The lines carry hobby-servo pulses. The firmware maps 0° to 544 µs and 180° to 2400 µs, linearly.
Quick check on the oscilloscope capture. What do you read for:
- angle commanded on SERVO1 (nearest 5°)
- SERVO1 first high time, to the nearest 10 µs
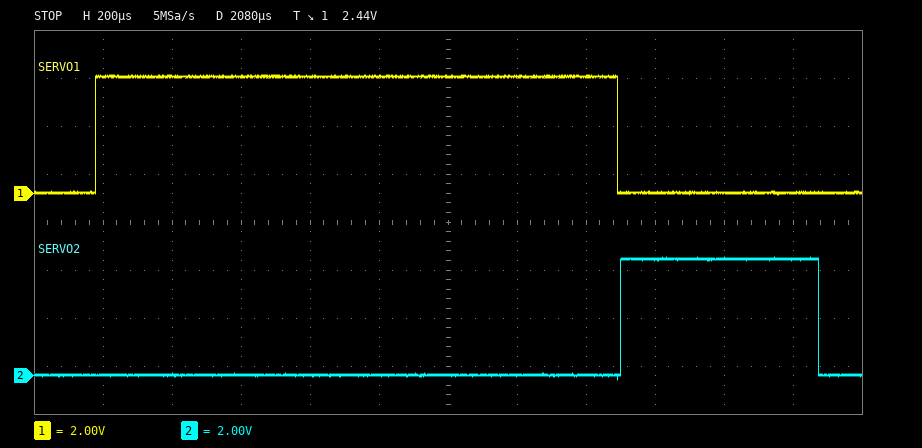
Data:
95°
1510 µs
